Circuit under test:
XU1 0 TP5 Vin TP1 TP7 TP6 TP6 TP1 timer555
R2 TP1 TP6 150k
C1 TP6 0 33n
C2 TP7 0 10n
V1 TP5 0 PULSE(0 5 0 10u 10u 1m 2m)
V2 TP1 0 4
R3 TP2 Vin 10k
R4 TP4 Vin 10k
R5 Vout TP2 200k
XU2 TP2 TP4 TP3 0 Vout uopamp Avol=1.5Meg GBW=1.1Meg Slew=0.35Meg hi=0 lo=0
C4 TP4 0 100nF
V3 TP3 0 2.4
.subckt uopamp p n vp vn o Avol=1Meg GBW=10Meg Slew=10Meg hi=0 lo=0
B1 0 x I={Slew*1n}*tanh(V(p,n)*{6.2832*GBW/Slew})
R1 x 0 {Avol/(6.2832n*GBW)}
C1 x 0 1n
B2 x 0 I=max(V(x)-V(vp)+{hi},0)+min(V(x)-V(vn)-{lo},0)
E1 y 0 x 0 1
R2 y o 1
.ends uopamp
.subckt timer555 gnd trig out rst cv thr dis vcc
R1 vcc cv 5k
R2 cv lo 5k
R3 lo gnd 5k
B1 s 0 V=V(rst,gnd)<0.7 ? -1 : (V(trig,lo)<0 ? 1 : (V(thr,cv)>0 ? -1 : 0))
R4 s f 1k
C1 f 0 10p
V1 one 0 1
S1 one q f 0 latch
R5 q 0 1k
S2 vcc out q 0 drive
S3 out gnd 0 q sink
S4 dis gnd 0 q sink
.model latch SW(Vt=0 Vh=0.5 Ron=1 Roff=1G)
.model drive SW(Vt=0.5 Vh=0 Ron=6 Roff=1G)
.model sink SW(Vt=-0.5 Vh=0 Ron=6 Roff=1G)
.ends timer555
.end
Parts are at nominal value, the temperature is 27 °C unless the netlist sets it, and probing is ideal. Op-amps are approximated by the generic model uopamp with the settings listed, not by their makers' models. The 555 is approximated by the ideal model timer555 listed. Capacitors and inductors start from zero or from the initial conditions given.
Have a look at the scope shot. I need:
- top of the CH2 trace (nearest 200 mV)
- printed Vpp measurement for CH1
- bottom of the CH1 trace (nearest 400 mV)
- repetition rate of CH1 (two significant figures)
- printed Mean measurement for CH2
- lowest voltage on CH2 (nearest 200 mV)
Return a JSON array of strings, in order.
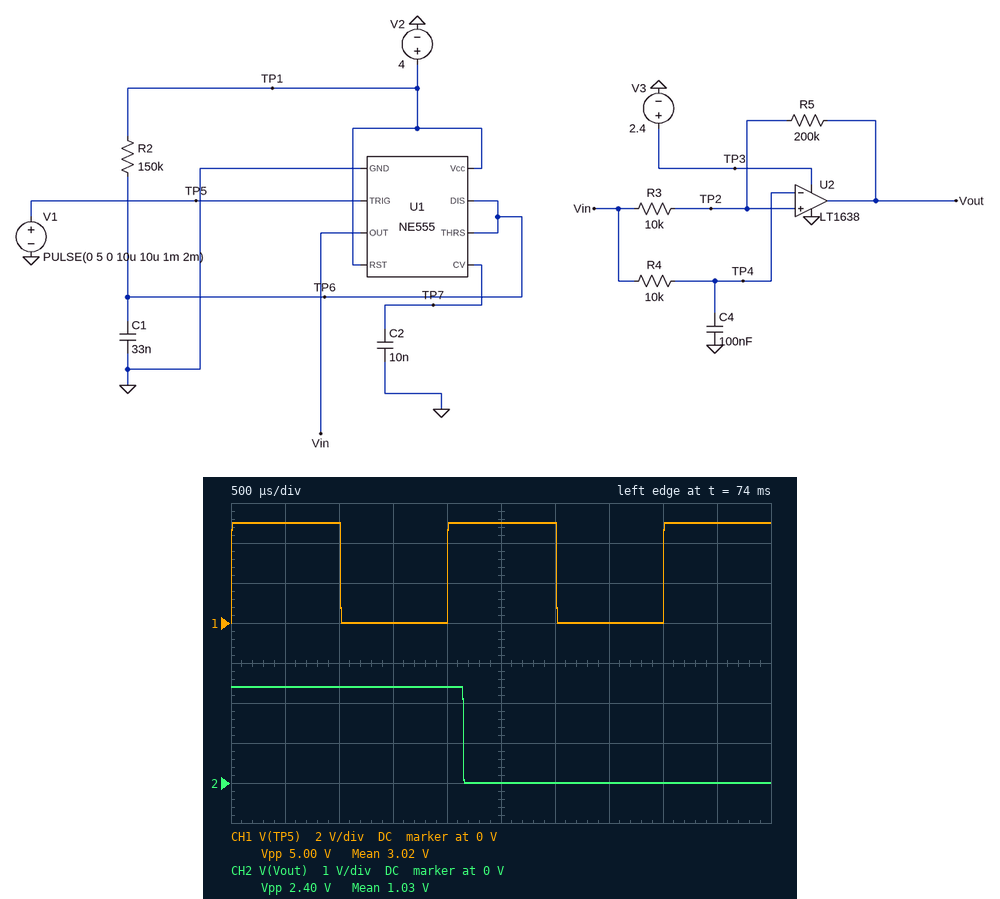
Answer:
["2.4 V", "5.00 V", "0 V", "500 Hz", "1.03 V", "0 V"]
